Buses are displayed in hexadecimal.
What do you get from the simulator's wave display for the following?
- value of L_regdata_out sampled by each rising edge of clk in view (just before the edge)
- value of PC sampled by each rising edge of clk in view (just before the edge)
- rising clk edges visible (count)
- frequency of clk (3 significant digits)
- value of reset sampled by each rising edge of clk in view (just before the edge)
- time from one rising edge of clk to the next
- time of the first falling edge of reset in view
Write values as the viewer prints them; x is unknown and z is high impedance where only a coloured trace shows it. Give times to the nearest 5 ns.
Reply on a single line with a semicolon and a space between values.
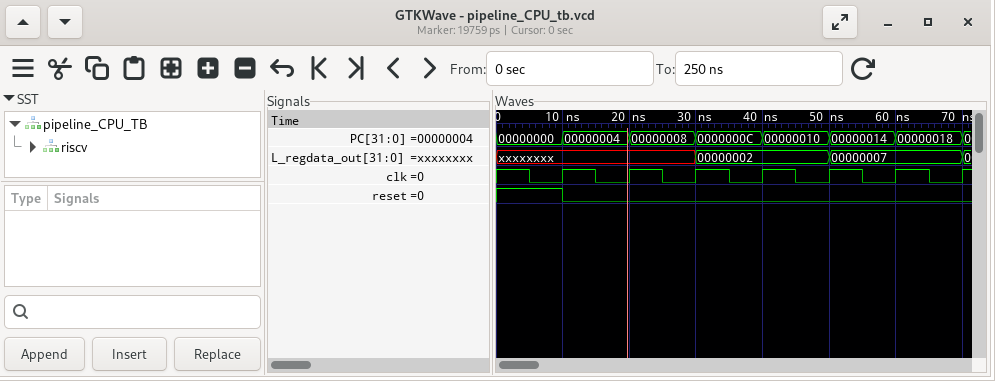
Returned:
xxxxxxxx, xxxxxxxx, xxxxxxxx, 00000002, 00000002, 00000007, 00000007; 00000000, 00000004, 00000008, 0000000C, 00000010, 00000014, 00000018; 7; 100 MHz; 1 0 0 0 0 0 0; 10 ns; 10 ns
